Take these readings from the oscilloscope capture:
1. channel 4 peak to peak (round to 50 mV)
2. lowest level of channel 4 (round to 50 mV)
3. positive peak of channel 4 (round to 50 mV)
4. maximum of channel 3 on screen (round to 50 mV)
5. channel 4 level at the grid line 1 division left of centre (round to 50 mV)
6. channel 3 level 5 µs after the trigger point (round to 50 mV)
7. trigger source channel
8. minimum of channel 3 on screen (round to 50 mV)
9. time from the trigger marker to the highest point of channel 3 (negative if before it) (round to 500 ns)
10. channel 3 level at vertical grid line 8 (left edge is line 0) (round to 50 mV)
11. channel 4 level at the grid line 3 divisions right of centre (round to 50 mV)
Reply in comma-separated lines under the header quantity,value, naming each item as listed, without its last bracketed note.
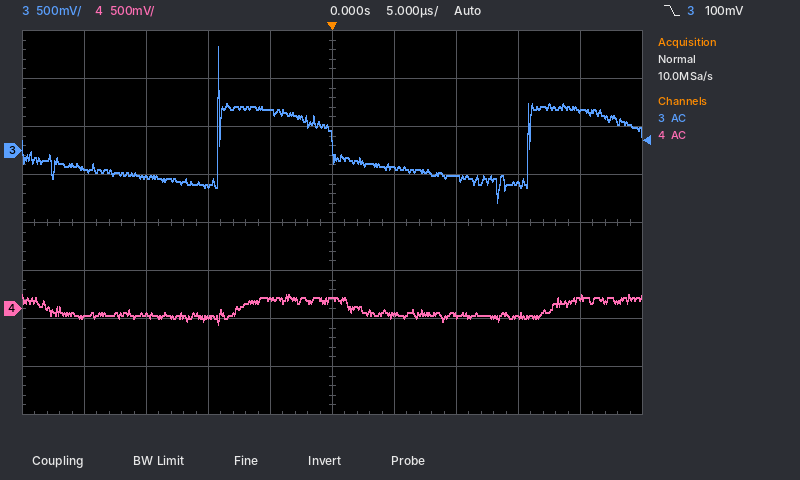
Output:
quantity,value
channel 4 peak to peak,300 mV
lowest level of channel 4,-150 mV
positive peak of channel 4,150 mV
maximum of channel 3 on screen,1.10 V
channel 4 level at the grid line 1 division left of centre,100 mV
channel 3 level 5 µs after the trigger point,-200 mV
trigger source channel,channel 3
minimum of channel 3 on screen,-550 mV
time from the trigger marker to the highest point of channel 3 (negative if before it),-9.0 µs
channel 3 level at vertical grid line 8 (left edge is line 0),-350 mV
channel 4 level at the grid line 3 divisions right of centre,-50 mV
